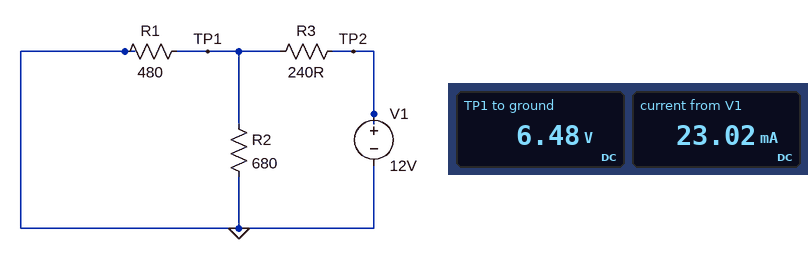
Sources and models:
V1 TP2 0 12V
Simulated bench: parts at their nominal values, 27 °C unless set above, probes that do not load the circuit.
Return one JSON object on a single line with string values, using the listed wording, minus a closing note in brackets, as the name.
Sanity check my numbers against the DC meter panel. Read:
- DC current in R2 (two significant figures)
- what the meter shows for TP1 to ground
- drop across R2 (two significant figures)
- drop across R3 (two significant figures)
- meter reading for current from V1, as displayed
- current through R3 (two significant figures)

{"DC current in R2": "9.5 mA", "what the meter shows for TP1 to ground": "6.48 V", "drop across R2": "6.5 V", "drop across R3": "5.5 V", "meter reading for current from V1, as displayed": "23.02 mA", "current through R3": "23 mA"}
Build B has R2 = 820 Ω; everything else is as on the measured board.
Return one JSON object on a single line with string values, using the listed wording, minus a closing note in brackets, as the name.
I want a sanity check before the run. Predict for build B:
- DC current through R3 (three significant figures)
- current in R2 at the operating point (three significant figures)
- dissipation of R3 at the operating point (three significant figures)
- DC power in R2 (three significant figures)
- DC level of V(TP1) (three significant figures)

{"DC current through R3": "22.1 mA", "current in R2 at the operating point": "8.16 mA", "dissipation of R3 at the operating point": "117 mW", "DC power in R2": "54.6 mW", "DC level of V(TP1)": "6.69 V"}
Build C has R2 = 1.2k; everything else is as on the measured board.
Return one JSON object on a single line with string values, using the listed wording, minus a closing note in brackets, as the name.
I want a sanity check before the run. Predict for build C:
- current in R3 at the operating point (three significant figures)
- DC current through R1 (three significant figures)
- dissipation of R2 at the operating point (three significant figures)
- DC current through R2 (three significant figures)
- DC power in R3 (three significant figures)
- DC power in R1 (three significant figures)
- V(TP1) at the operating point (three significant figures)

{"current in R3 at the operating point": "20.6 mA", "DC current through R1": "14.7 mA", "dissipation of R2 at the operating point": "41.5 mW", "DC current through R2": "5.88 mA", "DC power in R3": "102 mW", "DC power in R1": "104 mW", "V(TP1) at the operating point": "7.06 V"}
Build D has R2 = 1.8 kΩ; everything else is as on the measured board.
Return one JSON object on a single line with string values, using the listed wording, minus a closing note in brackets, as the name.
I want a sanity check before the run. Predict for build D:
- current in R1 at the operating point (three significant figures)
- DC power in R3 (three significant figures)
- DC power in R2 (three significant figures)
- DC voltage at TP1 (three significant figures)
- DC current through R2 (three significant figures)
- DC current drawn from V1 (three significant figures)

{"current in R1 at the operating point": "15.3 mA", "DC power in R3": "90.2 mW", "DC power in R2": "30.0 mW", "DC voltage at TP1": "7.35 V", "DC current through R2": "4.08 mA", "DC current drawn from V1": "19.4 mA"}
